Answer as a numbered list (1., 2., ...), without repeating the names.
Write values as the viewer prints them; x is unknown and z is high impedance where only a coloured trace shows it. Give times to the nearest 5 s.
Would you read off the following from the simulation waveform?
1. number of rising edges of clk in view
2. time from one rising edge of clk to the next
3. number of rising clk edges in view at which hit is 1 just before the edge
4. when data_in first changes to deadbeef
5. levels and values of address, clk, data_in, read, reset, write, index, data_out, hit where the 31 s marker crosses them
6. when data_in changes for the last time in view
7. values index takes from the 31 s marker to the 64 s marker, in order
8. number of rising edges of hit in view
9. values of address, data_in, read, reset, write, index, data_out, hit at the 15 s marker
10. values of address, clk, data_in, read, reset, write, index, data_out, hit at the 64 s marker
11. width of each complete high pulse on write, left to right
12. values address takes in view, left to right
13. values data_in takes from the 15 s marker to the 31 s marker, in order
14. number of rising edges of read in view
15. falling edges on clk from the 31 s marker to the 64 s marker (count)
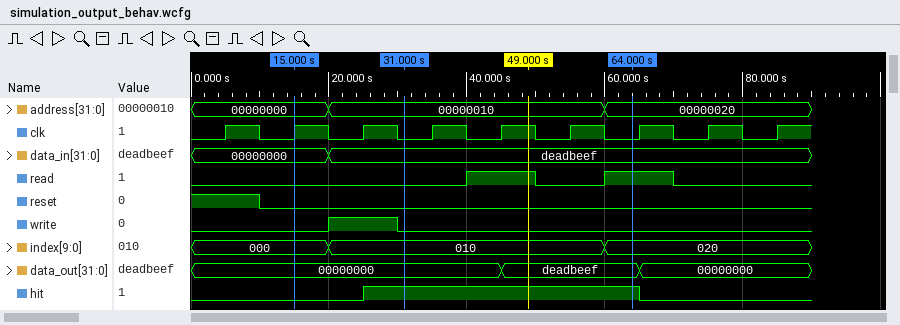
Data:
1. 9
2. 10 s
3. 4
4. 20 s
5. address=00000010, clk=0, data_in=deadbeef, read=0, reset=0, write=0, index=010, data_out=00000000, hit=1
6. 20 s
7. 010, 020
8. 1
9. address=00000000, data_in=00000000, read=0, reset=0, write=0, index=000, data_out=00000000, hit=0
10. address=00000020, clk=0, data_in=deadbeef, read=1, reset=0, write=0, index=020, data_out=deadbeef, hit=1
11. 10 s
12. 00000000, 00000010, 00000020
13. 00000000, deadbeef
14. 2
15. 3
